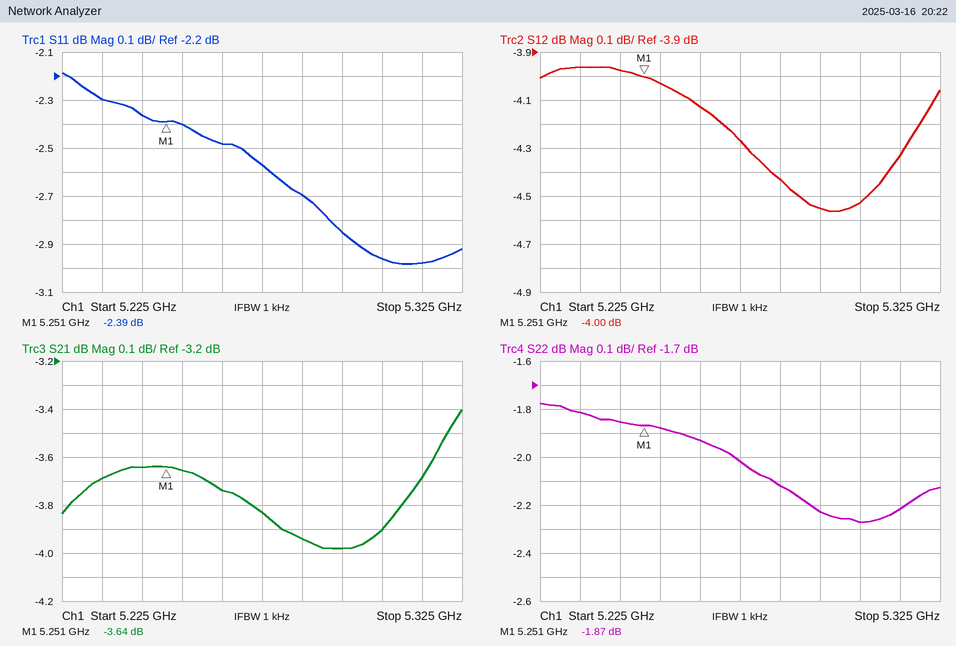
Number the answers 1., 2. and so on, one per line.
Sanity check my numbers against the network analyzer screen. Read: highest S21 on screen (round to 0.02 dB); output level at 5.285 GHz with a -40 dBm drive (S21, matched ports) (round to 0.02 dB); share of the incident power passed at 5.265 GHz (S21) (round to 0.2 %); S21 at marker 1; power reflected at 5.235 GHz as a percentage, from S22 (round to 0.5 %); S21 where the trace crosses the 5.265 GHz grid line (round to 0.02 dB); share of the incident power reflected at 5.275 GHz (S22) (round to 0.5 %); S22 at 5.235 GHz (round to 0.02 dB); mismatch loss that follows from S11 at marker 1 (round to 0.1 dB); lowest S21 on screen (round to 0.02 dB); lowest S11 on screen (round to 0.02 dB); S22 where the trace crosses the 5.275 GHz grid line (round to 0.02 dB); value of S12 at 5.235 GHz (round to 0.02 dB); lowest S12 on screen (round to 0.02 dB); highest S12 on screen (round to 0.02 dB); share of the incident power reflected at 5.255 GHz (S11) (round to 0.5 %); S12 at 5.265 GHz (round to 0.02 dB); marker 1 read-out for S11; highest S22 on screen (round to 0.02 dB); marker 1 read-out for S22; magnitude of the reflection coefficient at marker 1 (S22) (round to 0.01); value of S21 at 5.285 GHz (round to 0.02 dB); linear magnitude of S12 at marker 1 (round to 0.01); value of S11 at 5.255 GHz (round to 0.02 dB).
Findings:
1. -3.40 dB
2. -43.94 dBm
3. 42.2 %
4. -3.64 dB
5. 66.0 %
6. -3.74 dB
7. 63.0 %
8. -1.82 dB
9. 3.7 dB
10. -3.98 dB
11. -2.98 dB
12. -2.02 dB
13. -3.96 dB
14. -4.56 dB
15. -3.96 dB
16. 57.5 %
17. -4.12 dB
18. -2.39 dB
19. -1.78 dB
20. -1.87 dB
21. 0.81
22. -3.94 dB
23. 0.63
24. -2.40 dB
